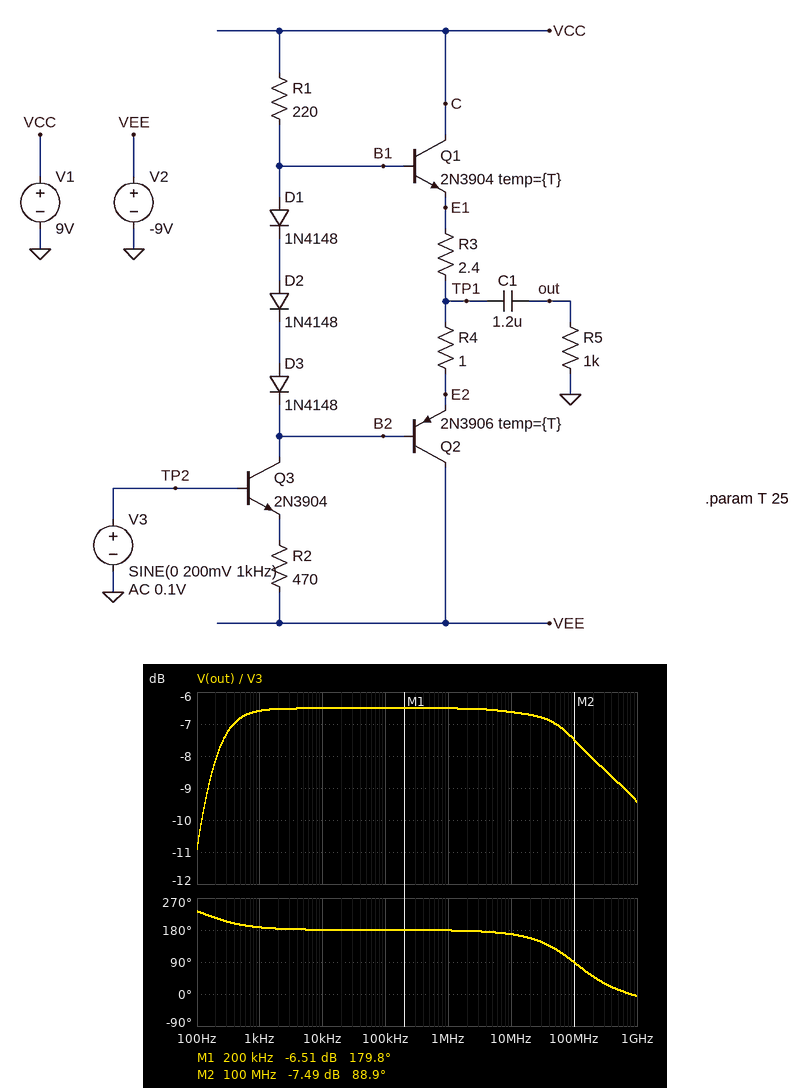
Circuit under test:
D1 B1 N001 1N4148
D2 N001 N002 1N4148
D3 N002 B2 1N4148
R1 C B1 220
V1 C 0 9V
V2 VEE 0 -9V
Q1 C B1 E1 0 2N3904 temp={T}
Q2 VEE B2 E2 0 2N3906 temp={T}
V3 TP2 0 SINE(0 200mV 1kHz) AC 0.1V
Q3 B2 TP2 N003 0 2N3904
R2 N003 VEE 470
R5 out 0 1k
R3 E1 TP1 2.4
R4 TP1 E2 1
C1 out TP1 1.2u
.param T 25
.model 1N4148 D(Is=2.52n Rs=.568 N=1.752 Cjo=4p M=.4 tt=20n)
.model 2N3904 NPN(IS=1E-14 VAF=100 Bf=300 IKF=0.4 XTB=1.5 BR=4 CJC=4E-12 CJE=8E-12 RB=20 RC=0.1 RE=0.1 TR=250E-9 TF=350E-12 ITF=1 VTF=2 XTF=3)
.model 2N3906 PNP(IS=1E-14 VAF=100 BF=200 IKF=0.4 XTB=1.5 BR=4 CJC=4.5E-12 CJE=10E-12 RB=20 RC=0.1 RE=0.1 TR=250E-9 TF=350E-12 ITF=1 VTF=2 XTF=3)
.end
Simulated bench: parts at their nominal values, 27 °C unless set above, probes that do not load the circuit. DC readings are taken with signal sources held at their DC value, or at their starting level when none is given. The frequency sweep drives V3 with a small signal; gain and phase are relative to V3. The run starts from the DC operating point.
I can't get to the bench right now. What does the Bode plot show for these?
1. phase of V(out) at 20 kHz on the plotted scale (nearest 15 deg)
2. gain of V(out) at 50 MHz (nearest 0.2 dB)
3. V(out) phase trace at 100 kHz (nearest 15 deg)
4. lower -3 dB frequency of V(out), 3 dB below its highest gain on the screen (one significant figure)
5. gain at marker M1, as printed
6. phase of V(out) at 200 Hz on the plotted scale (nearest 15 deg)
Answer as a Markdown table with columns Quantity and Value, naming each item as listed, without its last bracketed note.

| Quantity | Value |
|---|---|
| phase of V(out) at 20 kHz on the plotted scale | 180 deg |
| gain of V(out) at 50 MHz | -7.0 dB |
| V(out) phase trace at 100 kHz | 180 deg |
| lower -3 dB frequency of V(out), 3 dB below its highest gain on the screen | 100 Hz |
| gain at marker M1, as printed | -6.51 dB |
| phase of V(out) at 200 Hz on the plotted scale | 210 deg |
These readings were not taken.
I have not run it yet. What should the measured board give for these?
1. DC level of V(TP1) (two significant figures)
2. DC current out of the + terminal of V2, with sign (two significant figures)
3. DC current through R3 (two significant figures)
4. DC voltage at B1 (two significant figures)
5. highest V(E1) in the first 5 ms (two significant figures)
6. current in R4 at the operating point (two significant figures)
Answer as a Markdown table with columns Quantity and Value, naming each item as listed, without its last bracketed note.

| Quantity | Value |
|---|---|
| DC level of V(TP1) | 4.0 V |
| DC current out of the + terminal of V2, with sign | -170 mA |
| DC current through R3 | 150 mA |
| DC voltage at B1 | 5.2 V |
| highest V(E1) in the first 5 ms | 4.5 V |
| current in R4 at the operating point | 150 mA |
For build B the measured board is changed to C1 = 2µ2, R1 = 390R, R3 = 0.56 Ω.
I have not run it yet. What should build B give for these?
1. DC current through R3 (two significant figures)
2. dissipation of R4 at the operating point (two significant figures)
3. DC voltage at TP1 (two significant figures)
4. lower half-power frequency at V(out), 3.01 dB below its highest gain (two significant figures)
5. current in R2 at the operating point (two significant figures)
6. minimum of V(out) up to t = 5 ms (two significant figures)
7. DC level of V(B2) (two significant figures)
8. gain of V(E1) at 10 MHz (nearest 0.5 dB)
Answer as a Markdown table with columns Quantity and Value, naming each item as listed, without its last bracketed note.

| Quantity | Value |
|---|---|
| DC current through R3 | 260 mA |
| dissipation of R4 at the operating point | 69 mW |
| DC voltage at TP1 | 1.4 V |
| lower half-power frequency at V(out), 3.01 dB below its highest gain | 72 Hz |
| current in R2 at the operating point | 18 mA |
| minimum of V(out) up to t = 5 ms | -160 mV |
| DC level of V(B2) | 240 mV |
| gain of V(E1) at 10 MHz | -2.0 dB |
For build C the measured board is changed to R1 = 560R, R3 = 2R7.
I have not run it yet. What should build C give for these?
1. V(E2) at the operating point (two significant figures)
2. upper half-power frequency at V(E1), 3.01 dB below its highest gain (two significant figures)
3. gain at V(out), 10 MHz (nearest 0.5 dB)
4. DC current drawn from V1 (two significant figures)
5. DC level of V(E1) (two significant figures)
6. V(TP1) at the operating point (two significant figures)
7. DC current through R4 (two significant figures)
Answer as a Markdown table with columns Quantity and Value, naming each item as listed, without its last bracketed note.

| Quantity | Value |
|---|---|
| V(E2) at the operating point | 28 mV |
| upper half-power frequency at V(E1), 3.01 dB below its highest gain | 1.4 GHz |
| gain at V(out), 10 MHz | -0.5 dB |
| DC current drawn from V1 | 150 mA |
| DC level of V(E1) | 520 mV |
| V(TP1) at the operating point | 160 mV |
| DC current through R4 | 130 mA |
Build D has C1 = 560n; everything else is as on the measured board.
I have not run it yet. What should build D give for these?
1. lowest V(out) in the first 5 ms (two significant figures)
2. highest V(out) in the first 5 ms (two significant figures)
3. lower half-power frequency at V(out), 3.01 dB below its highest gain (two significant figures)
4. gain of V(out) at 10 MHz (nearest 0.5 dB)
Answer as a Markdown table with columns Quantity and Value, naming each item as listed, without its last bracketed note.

| Quantity | Value |
|---|---|
| lowest V(out) in the first 5 ms | -91 mV |
| highest V(out) in the first 5 ms | 98 mV |
| lower half-power frequency at V(out), 3.01 dB below its highest gain | 280 Hz |
| gain of V(out) at 10 MHz | -6.5 dB |
